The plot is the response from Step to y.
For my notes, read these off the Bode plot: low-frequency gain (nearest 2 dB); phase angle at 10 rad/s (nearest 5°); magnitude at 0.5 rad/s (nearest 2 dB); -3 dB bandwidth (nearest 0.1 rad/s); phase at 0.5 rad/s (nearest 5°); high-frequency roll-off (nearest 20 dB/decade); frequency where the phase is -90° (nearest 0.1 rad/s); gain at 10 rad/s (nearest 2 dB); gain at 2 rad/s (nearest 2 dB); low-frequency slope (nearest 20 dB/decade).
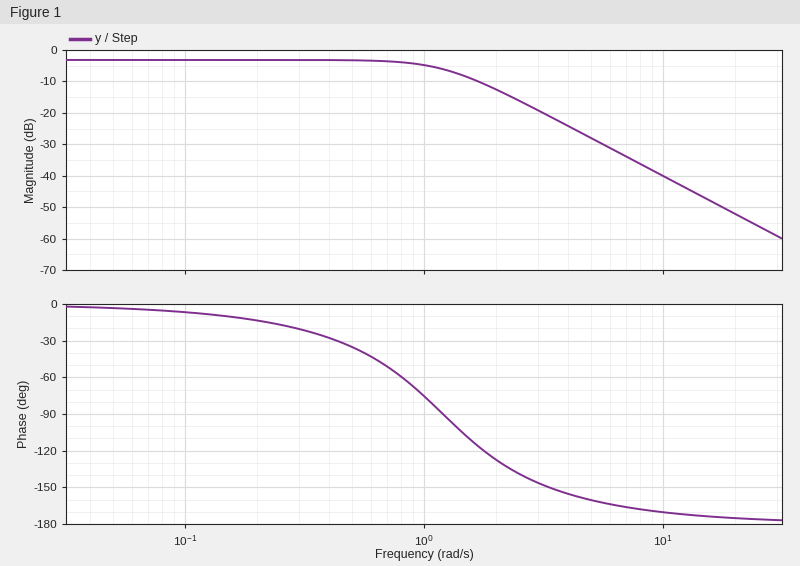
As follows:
-4 dB
-170°
-4 dB
1.2 rad/s
-35°
-40 dB/decade
1.2 rad/s
-40 dB
-12 dB
0 dB/decade
